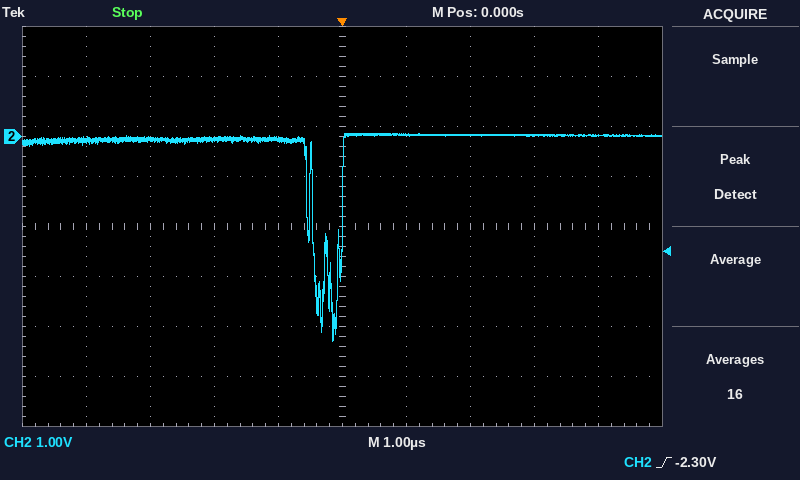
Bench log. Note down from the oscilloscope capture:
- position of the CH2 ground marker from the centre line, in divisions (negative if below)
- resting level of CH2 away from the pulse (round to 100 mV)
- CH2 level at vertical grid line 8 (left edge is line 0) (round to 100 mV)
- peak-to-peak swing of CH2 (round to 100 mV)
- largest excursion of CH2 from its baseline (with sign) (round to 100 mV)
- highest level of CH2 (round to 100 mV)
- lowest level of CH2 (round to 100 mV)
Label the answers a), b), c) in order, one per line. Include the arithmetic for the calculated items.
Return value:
a) +1.8 div
b) 0.0 V
c) 0.0 V
d) 100 mV − (-4.1 V) = 4.2 V
e) -4.1 V − (0.0 V) = -4.1 V
f) 100 mV
g) -4.1 V
